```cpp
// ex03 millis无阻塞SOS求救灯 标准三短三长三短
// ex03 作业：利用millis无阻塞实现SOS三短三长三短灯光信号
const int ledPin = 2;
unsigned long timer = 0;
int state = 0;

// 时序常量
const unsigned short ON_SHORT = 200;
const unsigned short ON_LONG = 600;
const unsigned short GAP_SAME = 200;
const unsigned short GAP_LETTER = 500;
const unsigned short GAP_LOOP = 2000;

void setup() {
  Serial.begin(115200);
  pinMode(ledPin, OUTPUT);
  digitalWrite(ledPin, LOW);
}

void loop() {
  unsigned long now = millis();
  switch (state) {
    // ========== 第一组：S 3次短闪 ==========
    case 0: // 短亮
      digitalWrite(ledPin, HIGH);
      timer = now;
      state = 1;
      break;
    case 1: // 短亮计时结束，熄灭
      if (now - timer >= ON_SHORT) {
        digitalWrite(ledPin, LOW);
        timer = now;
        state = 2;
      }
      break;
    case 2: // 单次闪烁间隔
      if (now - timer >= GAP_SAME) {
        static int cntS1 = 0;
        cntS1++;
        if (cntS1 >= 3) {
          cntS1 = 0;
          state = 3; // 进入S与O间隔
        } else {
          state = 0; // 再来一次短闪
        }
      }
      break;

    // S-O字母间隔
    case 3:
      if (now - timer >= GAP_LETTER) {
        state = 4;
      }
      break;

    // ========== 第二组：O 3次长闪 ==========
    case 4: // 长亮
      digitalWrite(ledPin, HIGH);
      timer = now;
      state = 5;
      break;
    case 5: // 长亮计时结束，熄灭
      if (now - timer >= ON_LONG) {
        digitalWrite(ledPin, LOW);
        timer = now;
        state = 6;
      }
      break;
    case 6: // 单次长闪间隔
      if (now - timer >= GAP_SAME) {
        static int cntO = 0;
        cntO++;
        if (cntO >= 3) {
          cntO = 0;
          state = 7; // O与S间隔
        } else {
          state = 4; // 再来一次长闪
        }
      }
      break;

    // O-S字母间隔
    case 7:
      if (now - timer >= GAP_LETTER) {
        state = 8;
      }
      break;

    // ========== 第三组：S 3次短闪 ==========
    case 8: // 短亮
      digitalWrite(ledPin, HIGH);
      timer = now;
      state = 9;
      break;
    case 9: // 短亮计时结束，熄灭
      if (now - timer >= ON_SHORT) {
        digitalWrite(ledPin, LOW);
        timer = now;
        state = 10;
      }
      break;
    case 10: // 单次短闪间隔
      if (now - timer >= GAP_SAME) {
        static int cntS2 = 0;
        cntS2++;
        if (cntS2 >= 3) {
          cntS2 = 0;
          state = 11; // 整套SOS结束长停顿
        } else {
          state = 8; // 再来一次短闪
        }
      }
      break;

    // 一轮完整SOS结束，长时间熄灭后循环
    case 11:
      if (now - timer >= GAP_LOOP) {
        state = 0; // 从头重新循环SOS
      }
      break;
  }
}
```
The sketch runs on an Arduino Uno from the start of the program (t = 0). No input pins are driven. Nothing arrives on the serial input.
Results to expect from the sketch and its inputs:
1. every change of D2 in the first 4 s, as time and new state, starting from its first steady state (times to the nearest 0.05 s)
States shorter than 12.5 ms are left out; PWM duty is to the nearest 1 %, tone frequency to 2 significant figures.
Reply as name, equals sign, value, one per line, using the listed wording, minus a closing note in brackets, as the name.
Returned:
every change of D2 in the first 4 s, as time and new state, starting from its first steady state = 0 s high; 0.2 s low; 0.4 s high; 0.6 s low; 0.8 s high; 1 s low; 1.5 s high; 2.1 s low; 2.3 s high; 2.9 s low; 3.1 s high; 3.7 s low
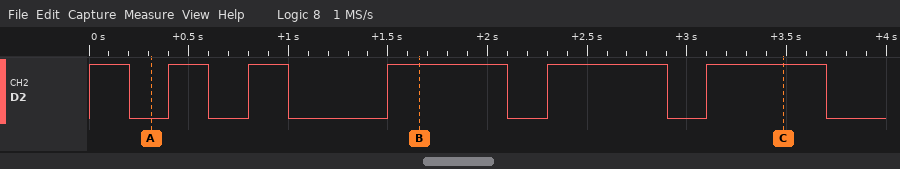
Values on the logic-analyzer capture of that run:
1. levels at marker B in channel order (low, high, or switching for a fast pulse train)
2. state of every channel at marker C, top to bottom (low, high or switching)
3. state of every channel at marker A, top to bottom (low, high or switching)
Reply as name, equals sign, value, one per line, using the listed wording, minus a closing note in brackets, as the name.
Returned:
levels at marker B in channel order = D2 high
state of every channel at marker C, top to bottom = D2 high
state of every channel at marker A, top to bottom = D2 low
